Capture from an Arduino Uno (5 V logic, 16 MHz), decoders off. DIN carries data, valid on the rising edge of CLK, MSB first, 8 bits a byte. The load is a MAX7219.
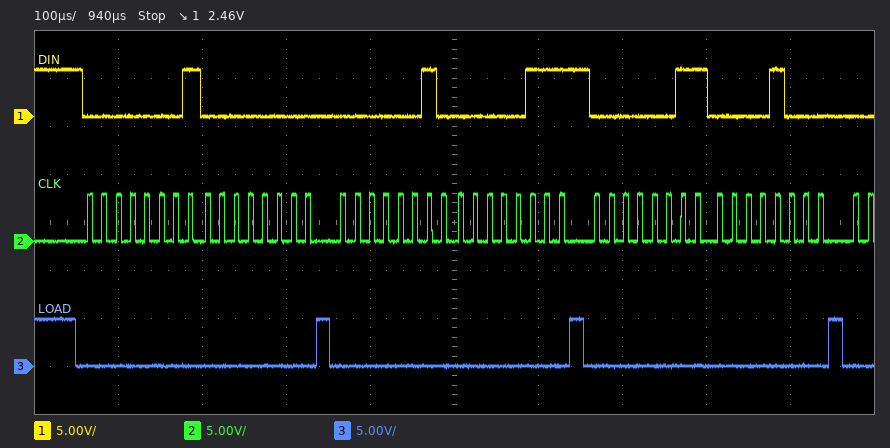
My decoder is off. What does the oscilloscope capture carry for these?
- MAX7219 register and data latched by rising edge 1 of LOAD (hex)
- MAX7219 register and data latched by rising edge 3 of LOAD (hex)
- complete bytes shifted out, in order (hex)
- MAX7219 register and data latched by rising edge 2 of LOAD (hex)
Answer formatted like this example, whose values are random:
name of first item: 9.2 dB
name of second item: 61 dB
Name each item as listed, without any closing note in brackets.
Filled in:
MAX7219 register and data latched by rising edge 1 of LOAD: register 0x1, data 0x00
MAX7219 register and data latched by rising edge 3 of LOAD: register 0x3, data 0x08
complete bytes shifted out, in order: 01 00 02 07 03 08
MAX7219 register and data latched by rising edge 2 of LOAD: register 0x2, data 0x07
